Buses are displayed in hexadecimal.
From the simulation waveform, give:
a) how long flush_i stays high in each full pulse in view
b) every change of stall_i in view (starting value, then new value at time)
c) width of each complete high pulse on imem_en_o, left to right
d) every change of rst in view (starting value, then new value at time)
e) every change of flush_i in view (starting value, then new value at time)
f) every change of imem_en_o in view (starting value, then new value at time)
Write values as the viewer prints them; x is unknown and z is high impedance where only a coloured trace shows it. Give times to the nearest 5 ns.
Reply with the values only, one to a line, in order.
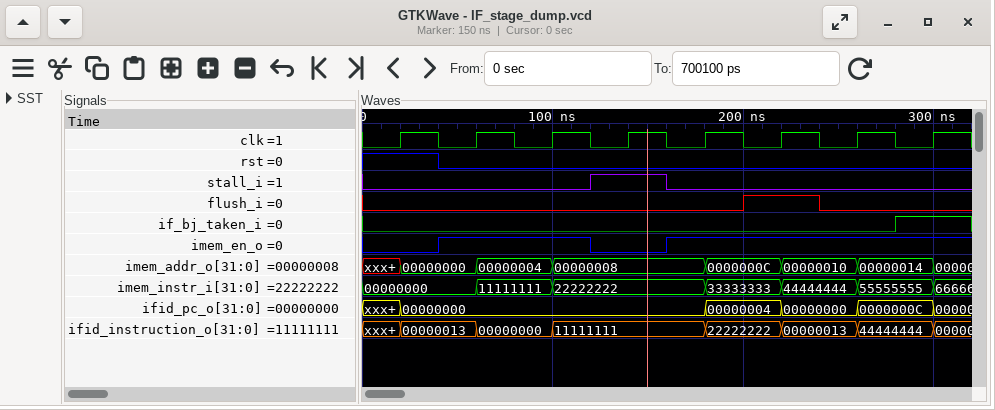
40 ns
0, 1 at 120 ns, 0 at 160 ns
80 ns
1, 0 at 40 ns
0, 1 at 200 ns, 0 at 240 ns
0, 1 at 40 ns, 0 at 120 ns, 1 at 160 ns
